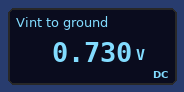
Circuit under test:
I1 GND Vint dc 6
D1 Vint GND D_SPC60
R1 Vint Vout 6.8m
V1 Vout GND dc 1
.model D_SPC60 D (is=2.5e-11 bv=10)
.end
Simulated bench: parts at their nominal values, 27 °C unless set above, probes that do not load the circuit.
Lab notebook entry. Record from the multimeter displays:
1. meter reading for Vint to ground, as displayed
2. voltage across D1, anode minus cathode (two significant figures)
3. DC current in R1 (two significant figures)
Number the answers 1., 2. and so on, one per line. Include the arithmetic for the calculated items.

1. 0.730 V
2. 730 mV = 730 mV
3. (1 V - 730 mV) / 6.8 mΩ = 40 A
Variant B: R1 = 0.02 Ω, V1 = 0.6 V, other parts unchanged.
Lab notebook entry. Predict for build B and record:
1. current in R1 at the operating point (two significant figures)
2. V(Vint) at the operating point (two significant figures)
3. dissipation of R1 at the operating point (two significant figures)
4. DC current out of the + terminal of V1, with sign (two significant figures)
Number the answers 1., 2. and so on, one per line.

1. 3.0 A
2. 660 mV
3. 180 mW
4. -3.0 A
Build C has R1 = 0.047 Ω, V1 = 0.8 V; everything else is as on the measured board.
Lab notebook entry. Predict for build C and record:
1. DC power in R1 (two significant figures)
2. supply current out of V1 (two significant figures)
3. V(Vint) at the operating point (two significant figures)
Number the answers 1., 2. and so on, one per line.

1. 270 mW
2. 2.4 A
3. 690 mV
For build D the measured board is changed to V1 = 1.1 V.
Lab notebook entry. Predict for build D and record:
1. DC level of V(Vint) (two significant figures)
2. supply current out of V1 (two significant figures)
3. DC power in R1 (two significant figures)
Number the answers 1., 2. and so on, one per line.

1. 740 mV
2. 53 A
3. 19 W
